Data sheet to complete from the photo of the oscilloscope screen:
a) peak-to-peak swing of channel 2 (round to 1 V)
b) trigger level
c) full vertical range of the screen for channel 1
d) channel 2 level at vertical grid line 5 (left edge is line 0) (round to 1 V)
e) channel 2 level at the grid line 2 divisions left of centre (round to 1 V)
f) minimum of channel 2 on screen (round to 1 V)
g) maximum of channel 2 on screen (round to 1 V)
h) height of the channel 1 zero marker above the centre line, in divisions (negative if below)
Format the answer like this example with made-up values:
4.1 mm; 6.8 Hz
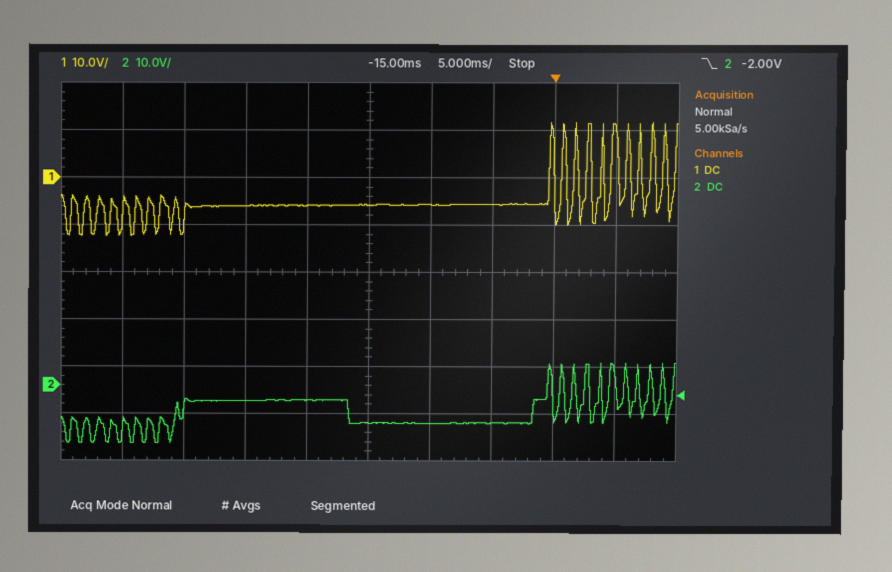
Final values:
17 V; -2.00 V; 80 V; -8 V; -3 V; -12 V; 5 V; +2.0 div
